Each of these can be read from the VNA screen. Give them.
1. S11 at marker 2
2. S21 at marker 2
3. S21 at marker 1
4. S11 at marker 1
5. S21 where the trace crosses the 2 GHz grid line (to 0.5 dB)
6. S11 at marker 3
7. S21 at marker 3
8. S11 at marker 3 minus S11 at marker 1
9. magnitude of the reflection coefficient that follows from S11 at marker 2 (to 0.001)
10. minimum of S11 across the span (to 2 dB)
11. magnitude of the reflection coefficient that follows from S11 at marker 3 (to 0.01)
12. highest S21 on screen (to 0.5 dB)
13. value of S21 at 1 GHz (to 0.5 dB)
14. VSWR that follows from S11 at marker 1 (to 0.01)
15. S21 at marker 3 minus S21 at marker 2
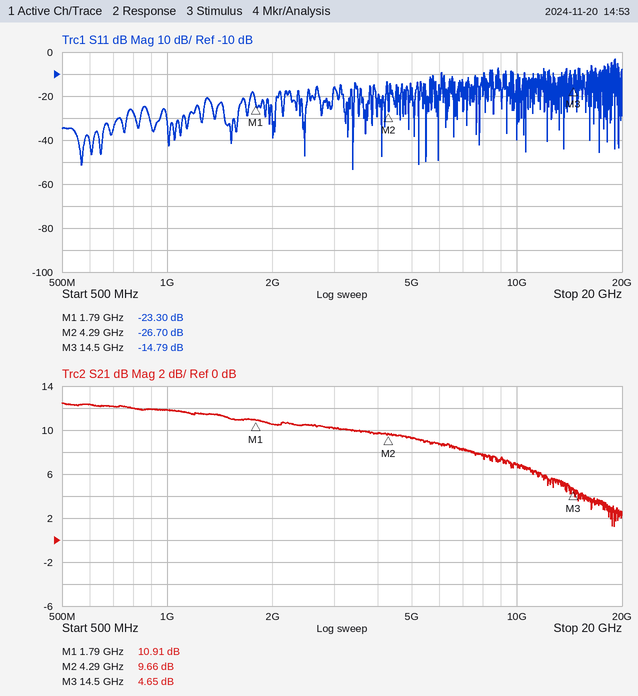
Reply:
-26.70 dB
9.66 dB
10.91 dB
-23.30 dB
10.5 dB
-14.79 dB
4.65 dB
8.51 dB
0.046
-54 dB
0.18
12.5 dB
12.0 dB
1.15
-5.01 dB
